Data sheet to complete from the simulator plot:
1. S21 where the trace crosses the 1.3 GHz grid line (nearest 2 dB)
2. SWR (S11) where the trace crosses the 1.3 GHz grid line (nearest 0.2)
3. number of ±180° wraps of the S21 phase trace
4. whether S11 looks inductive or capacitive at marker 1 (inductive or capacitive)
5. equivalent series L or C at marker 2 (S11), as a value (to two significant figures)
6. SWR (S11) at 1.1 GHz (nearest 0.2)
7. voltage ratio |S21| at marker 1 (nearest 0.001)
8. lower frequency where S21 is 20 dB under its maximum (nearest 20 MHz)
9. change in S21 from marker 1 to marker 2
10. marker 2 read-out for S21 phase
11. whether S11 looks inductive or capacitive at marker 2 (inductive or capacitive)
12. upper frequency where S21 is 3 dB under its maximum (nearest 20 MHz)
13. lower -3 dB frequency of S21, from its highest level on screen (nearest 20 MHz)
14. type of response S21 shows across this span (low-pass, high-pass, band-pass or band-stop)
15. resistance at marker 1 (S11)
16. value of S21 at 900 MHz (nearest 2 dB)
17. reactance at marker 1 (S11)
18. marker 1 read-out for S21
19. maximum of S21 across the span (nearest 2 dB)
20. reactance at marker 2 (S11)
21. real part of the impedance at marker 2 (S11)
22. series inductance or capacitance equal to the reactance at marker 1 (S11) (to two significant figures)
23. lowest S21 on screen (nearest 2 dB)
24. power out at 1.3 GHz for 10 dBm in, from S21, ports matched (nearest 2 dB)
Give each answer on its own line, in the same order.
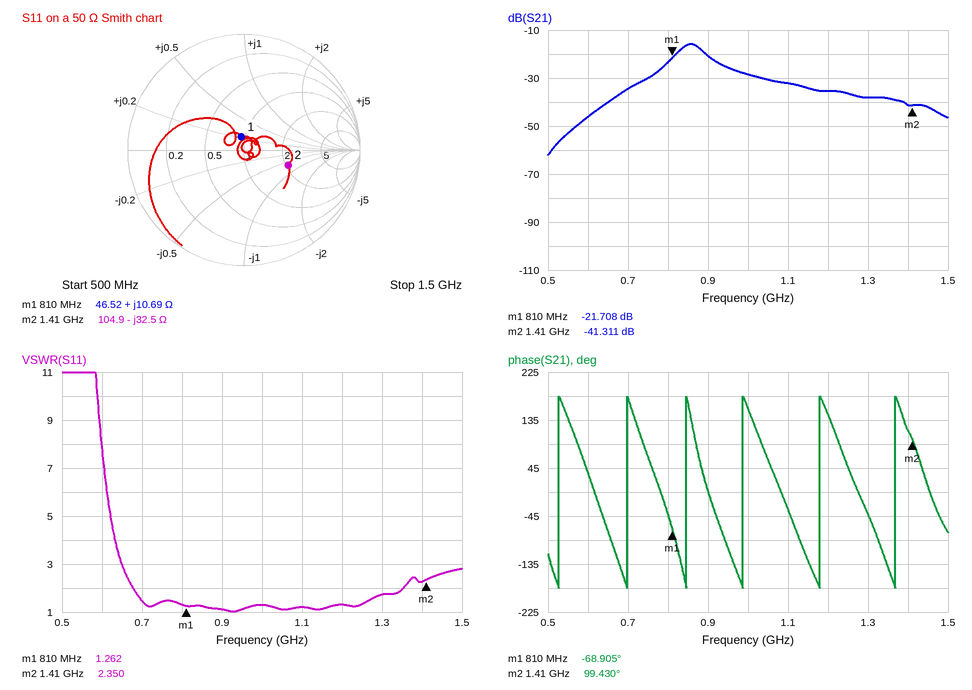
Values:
-38 dB
1.8
6
inductive
3.5 pF
1.2
0.082
680 MHz
-19.603 dB
99.430°
capacitive
880 MHz
820 MHz
band-pass
46.52 Ω
-20 dB
+10.69 Ω
-21.708 dB
-16 dB
-32.5 Ω
104.9 Ω
2.1 nH
-62 dB
-28 dBm
